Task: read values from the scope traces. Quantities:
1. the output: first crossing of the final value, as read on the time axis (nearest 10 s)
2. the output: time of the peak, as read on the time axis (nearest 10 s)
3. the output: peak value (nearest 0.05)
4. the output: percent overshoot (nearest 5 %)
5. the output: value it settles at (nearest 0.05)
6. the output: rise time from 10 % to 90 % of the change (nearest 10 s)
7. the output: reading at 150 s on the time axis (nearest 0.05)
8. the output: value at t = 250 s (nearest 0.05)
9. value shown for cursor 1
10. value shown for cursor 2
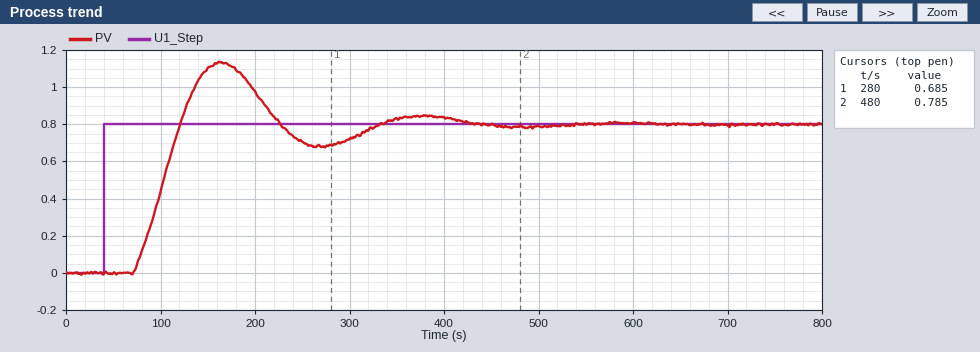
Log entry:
120 s
160 s
1.15
40 %
0.80
40 s
1.10
0.70
0.685
0.785
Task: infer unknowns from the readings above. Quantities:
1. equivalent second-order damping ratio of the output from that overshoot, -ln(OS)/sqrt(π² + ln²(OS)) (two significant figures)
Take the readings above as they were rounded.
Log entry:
0.28
